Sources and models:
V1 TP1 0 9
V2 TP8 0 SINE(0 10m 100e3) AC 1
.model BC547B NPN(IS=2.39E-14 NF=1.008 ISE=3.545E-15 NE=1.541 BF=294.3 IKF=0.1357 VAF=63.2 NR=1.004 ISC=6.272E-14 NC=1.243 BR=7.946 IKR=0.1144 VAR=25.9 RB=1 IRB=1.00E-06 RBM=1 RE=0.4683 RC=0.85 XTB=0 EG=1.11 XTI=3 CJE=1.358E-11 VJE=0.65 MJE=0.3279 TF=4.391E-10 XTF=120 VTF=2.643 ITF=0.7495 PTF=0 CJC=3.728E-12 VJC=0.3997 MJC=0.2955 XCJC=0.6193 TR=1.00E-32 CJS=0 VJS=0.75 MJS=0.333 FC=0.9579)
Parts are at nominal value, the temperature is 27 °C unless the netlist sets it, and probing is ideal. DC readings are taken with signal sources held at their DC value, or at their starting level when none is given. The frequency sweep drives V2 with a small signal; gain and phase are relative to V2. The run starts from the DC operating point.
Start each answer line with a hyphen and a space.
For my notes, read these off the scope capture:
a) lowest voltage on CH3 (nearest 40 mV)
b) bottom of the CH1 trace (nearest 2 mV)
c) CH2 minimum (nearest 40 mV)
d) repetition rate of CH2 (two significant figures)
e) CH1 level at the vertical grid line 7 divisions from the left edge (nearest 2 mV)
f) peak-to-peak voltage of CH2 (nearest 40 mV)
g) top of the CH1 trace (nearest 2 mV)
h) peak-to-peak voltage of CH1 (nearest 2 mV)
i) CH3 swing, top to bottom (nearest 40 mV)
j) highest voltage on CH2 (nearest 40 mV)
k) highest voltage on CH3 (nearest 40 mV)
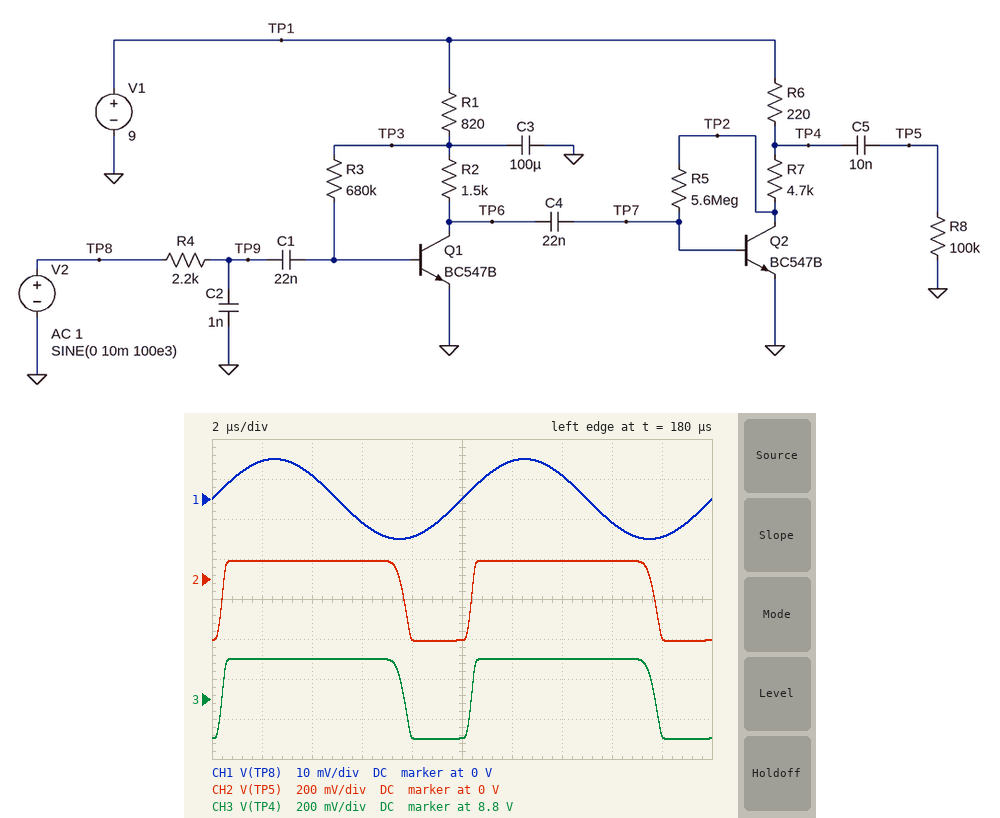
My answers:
- 8.60 V
- -10 mV
- -320 mV
- 100 kHz
- 6 mV
- 400 mV
- 10 mV
- 20 mV
- 400 mV
- 80 mV
- 9.00 V
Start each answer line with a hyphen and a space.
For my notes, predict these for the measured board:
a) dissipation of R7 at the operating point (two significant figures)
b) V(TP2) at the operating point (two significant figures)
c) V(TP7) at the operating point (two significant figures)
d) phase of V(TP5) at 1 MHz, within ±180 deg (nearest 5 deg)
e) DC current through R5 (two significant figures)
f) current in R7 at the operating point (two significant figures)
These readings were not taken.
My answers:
- 640 µW
- 7.2 V
- 610 mV
- -130 deg
- 1.2 µA
- 370 µA
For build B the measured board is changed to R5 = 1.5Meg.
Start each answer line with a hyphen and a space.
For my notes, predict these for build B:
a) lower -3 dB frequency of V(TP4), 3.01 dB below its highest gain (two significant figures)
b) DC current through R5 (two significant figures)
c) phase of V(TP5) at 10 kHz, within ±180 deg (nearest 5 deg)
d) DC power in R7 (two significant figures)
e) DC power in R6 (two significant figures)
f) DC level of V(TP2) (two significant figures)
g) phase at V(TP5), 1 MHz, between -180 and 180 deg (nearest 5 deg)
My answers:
- 1.9 kHz
- 2.8 µA
- 10 deg
- 3.4 mW
- 160 µW
- 4.8 V
- -145 deg
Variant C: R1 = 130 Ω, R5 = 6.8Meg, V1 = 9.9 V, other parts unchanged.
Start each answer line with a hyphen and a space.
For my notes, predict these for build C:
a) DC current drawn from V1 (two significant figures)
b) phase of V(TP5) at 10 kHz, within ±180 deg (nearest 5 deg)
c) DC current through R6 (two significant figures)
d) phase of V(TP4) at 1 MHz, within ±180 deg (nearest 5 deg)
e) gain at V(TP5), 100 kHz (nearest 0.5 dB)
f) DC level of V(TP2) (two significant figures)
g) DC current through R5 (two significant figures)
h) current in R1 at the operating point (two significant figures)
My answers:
- 4.1 mA
- 5 deg
- 350 µA
- -125 deg
- 44.5 dB
- 8.2 V
- 1.1 µA
- 3.8 mA
